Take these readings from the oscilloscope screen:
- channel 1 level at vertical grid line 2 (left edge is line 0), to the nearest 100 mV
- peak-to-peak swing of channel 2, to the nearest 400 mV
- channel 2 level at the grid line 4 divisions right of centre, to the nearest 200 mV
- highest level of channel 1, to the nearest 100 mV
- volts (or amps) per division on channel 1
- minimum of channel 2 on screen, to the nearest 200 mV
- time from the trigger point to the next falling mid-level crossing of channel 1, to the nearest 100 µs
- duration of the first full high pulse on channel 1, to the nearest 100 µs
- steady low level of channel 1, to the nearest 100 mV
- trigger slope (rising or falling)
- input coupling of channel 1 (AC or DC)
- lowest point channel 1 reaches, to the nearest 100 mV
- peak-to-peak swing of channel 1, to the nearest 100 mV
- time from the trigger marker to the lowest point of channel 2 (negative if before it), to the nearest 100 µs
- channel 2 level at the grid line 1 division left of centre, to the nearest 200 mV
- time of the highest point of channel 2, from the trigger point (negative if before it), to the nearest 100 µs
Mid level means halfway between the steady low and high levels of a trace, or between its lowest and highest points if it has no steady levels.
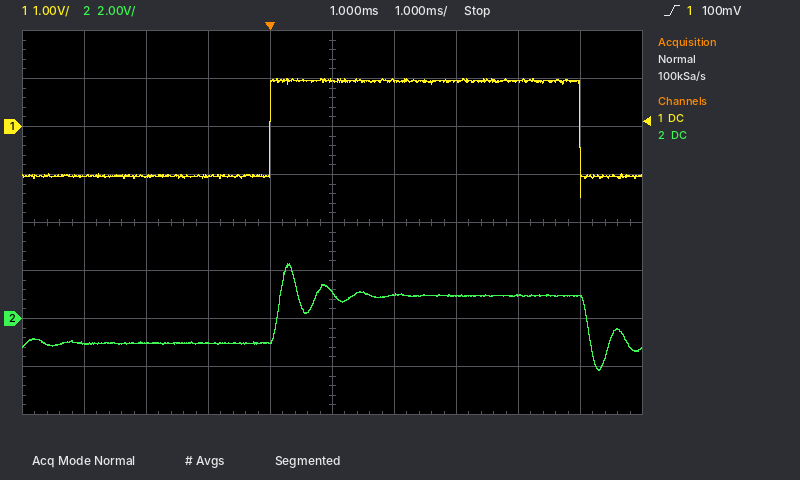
-1.0 V
4.4 V
800 mV
1.0 V
1 V
-2.2 V
5.0 ms
5.0 ms
-1.0 V
rising
DC
-1.5 V
2.5 V
+5.3 ms
-1.0 V
+300 µs
